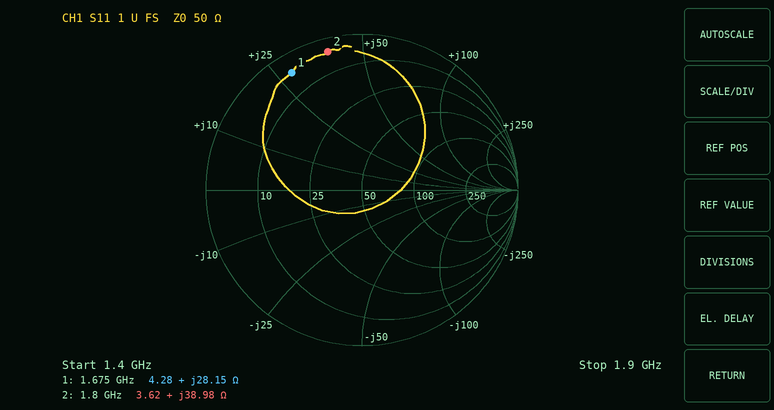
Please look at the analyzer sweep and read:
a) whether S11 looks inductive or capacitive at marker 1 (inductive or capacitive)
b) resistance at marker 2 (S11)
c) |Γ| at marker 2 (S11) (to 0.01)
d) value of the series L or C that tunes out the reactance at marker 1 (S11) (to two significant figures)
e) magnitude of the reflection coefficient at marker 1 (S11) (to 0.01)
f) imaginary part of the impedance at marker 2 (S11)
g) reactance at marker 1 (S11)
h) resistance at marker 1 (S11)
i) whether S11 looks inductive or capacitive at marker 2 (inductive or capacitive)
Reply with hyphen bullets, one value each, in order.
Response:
- inductive
- 3.62 Ω
- 0.91
- 3.4 pF
- 0.88
- +38.98 Ω
- +28.15 Ω
- 4.28 Ω
- inductive
